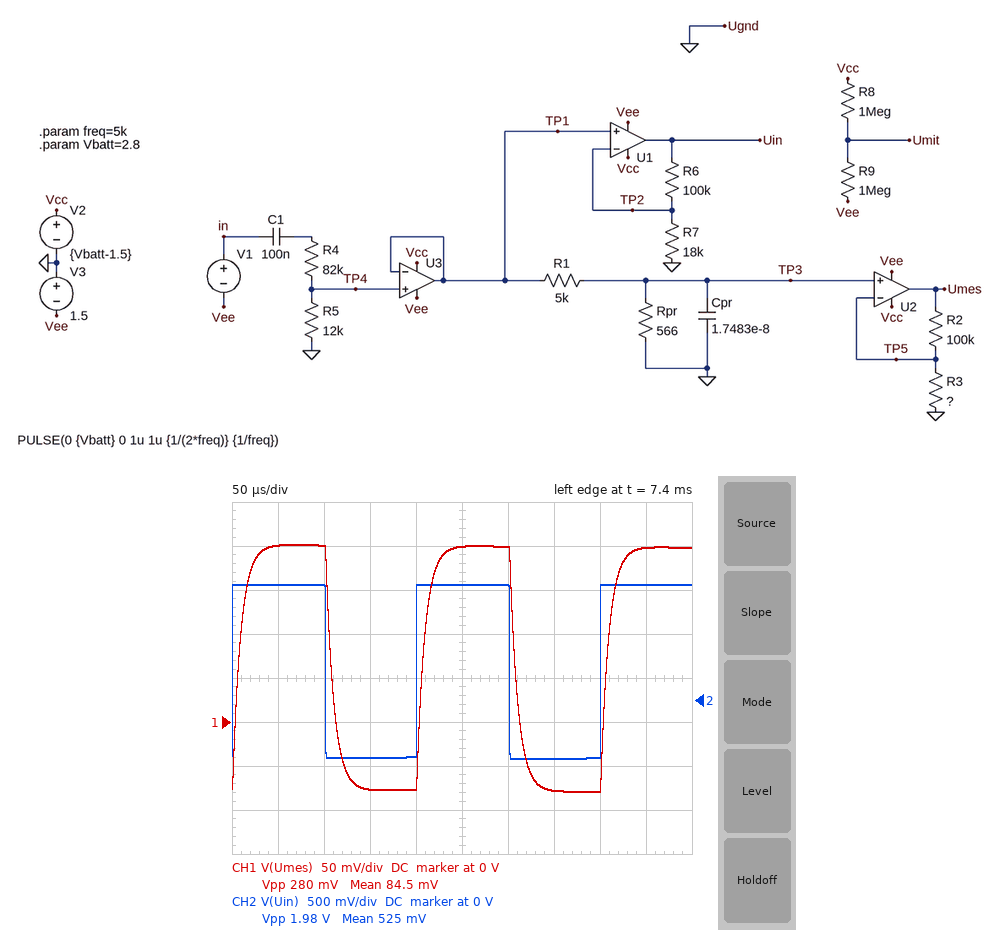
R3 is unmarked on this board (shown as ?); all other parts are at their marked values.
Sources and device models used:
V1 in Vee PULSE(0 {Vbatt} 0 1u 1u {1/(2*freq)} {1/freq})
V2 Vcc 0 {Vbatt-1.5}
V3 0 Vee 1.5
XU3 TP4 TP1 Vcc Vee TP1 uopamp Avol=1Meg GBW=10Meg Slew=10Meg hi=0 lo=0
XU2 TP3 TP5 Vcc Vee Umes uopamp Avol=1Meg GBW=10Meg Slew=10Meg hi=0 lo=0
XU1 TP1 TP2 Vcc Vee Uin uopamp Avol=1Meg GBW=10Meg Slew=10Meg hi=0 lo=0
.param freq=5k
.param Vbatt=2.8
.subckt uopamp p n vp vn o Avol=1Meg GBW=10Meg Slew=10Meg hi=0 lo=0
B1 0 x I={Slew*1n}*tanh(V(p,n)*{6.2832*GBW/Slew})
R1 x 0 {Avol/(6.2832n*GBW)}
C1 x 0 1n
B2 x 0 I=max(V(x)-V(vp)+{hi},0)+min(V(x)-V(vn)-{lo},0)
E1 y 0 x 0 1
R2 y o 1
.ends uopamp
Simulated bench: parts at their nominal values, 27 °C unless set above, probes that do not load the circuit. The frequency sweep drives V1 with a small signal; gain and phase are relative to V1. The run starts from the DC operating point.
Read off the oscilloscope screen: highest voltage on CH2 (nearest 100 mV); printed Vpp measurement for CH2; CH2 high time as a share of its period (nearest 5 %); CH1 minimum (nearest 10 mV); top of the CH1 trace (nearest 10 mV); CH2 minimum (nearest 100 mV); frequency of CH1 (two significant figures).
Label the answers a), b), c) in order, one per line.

a) 1.3 V
b) 1.98 V
c) 50 %
d) -80 mV
e) 200 mV
f) -700 mV
g) 5.0 kHz
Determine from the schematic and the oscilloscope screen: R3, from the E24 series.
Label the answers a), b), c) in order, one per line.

a) 15 kΩ
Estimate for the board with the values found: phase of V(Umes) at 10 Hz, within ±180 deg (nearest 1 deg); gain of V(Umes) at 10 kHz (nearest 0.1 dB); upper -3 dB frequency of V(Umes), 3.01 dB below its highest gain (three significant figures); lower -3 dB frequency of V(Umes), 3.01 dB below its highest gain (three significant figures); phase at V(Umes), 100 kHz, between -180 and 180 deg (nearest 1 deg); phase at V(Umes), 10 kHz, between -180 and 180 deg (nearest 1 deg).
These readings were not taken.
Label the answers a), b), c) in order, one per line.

a) 59 deg
b) -21.2 dB
c) 17.9 kHz
d) 16.9 Hz
e) -85 deg
f) -30 deg
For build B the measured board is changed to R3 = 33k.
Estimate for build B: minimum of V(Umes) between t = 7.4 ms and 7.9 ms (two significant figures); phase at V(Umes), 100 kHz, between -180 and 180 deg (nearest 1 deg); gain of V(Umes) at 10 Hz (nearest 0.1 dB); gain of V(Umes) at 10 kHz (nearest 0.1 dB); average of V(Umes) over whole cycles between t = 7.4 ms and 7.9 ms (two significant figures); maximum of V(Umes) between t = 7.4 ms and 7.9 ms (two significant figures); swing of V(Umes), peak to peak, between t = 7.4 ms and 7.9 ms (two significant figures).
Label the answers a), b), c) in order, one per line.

a) -42 mV
b) -83 deg
c) -31.5 dB
d) -26.8 dB
e) 33 mV
f) 110 mV
g) 150 mV
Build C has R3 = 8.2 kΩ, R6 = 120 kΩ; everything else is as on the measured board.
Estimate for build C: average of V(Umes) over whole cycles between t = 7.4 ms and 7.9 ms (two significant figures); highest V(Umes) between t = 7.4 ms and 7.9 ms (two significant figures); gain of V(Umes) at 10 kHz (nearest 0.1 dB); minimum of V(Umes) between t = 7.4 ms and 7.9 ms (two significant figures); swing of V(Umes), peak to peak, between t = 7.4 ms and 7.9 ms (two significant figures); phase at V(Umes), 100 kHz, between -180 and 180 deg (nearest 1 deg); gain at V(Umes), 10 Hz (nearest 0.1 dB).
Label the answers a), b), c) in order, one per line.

a) 110 mV
b) 350 mV
c) -16.5 dB
d) -140 mV
e) 480 mV
f) -88 deg
g) -21.2 dB
